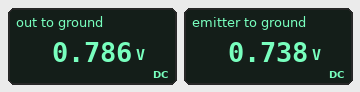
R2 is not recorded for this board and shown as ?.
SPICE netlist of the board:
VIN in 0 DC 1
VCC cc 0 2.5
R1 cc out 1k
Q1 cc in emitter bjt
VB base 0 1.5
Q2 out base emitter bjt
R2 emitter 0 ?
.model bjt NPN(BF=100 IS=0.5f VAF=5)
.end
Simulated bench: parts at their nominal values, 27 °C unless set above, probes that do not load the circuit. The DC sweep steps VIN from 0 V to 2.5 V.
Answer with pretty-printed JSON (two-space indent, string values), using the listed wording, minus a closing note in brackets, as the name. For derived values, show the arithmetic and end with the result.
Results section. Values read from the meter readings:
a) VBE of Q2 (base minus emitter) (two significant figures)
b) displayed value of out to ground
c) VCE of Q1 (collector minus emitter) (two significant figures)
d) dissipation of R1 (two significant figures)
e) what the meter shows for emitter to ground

{
  "VBE of Q2 (base minus emitter)": "1.5 V - 738 mV = 760 mV",
  "displayed value of out to ground": "0.786 V",
  "VCE of Q1 (collector minus emitter)": "2.5 V - 738 mV = 1.8 V",
  "dissipation of R1": "(2.5 V - 786 mV)^2 / 1 kΩ = 2.9 mW",
  "what the meter shows for emitter to ground": "0.738 V"
}
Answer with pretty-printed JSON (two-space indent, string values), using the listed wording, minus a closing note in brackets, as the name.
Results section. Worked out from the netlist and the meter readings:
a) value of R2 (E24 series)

{
  "value of R2": "330 Ω"
}
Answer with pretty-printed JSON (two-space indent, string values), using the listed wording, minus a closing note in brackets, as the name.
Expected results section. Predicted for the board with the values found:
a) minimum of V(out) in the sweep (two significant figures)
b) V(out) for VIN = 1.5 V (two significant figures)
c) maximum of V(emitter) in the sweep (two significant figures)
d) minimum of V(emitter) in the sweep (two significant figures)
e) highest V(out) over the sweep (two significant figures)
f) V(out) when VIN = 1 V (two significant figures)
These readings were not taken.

{
  "minimum of V(out) in the sweep": "790 mV",
  "V(out) for VIN = 1.5 V": "1.5 V",
  "maximum of V(emitter) in the sweep": "1.7 V",
  "minimum of V(emitter) in the sweep": "740 mV",
  "highest V(out) over the sweep": "2.5 V",
  "V(out) when VIN = 1 V": "790 mV"
}
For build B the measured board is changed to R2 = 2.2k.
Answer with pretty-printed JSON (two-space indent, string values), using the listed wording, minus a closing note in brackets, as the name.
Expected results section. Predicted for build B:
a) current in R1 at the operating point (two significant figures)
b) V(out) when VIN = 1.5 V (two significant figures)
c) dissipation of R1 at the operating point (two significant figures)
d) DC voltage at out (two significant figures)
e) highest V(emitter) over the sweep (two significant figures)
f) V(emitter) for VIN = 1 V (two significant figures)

{
  "current in R1 at the operating point": "360 µA",
  "V(out) when VIN = 1.5 V": "2.3 V",
  "dissipation of R1 at the operating point": "130 µW",
  "DC voltage at out": "2.1 V",
  "highest V(emitter) over the sweep": "1.8 V",
  "V(emitter) for VIN = 1 V": "800 mV"
}
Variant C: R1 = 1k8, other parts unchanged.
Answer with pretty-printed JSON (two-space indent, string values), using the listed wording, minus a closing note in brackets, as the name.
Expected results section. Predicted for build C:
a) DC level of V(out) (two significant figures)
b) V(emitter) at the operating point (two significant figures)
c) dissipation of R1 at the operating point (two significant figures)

{
  "DC level of V(out)": "760 mV",
  "V(emitter) at the operating point": "730 mV",
  "dissipation of R1 at the operating point": "1.7 mW"
}
